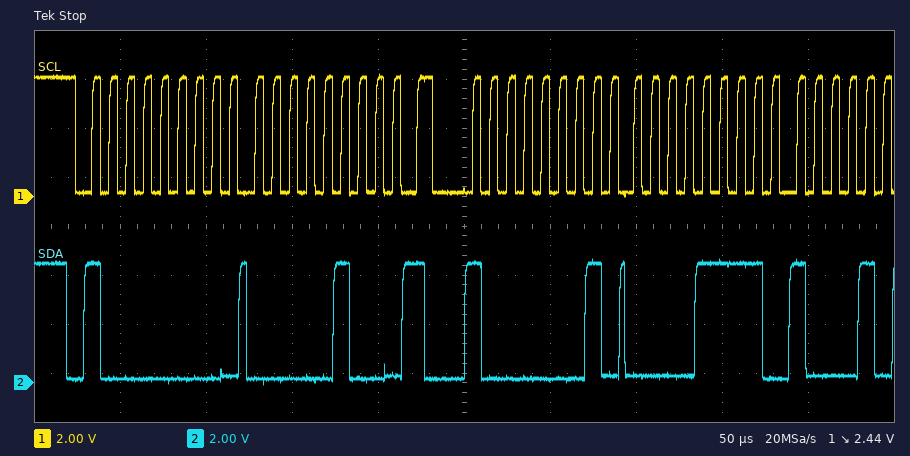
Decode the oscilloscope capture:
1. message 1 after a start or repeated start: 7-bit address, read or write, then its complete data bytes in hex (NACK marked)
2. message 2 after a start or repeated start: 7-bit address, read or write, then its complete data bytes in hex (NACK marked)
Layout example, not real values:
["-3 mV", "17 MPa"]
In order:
["0x40 write: 04", "0x40 read: 0F"]
